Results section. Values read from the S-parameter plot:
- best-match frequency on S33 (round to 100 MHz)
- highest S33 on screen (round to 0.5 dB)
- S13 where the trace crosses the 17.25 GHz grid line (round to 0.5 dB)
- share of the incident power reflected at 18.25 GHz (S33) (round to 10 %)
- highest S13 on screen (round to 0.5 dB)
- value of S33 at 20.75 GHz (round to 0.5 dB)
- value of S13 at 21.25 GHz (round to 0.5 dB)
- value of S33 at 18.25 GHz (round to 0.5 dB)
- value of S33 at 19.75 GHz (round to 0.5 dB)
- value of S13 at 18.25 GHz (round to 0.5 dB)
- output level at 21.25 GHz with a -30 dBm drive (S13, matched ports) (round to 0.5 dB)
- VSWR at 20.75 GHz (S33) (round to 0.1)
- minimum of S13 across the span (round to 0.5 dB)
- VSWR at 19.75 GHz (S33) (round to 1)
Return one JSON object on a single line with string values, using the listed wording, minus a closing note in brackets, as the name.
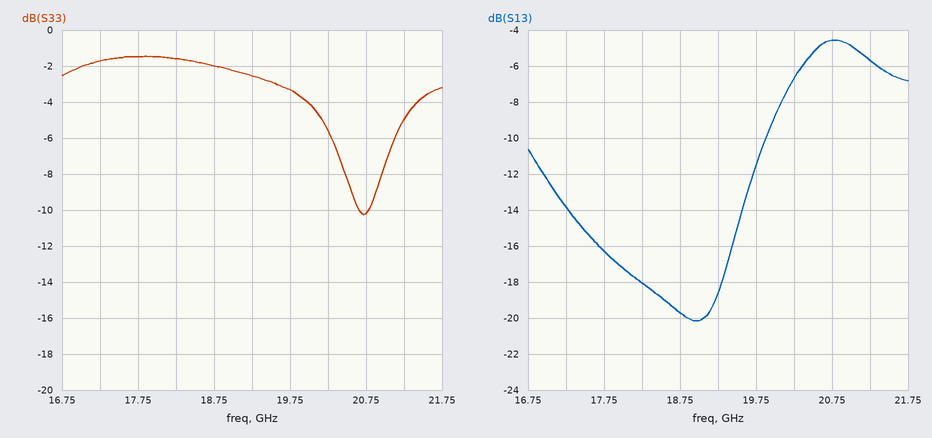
{"best-match frequency on S33": "20.7 GHz", "highest S33 on screen": "-1.5 dB", "S13 where the trace crosses the 17.25 GHz grid line": "-14.0 dB", "share of the incident power reflected at 18.25 GHz (S33)": "70 %", "highest S13 on screen": "-4.5 dB", "value of S33 at 20.75 GHz": "-10.0 dB", "value of S13 at 21.25 GHz": "-5.5 dB", "value of S33 at 18.25 GHz": "-1.5 dB", "value of S33 at 19.75 GHz": "-3.5 dB", "value of S13 at 18.25 GHz": "-18.0 dB", "output level at 21.25 GHz with a -30 dBm drive (S13, matched ports)": "-35.5 dBm", "VSWR at 20.75 GHz (S33)": "1.9", "minimum of S13 across the span": "-20.0 dB", "VSWR at 19.75 GHz (S33)": "5"}
